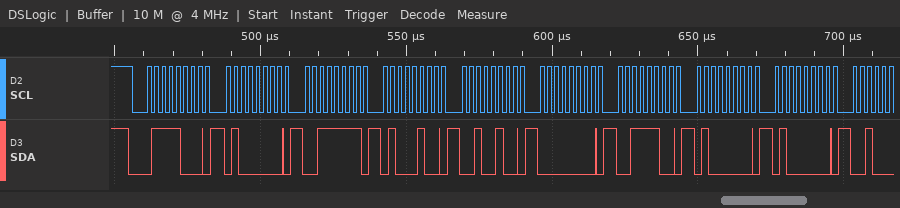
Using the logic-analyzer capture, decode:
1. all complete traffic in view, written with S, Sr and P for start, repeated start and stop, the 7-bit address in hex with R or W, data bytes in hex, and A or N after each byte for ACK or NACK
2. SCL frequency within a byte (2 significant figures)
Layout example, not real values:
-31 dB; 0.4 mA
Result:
S 3CW A 40 A 3F A 44 A 24 A 00 A 3C A 40 A 40 A; 400 kHz
